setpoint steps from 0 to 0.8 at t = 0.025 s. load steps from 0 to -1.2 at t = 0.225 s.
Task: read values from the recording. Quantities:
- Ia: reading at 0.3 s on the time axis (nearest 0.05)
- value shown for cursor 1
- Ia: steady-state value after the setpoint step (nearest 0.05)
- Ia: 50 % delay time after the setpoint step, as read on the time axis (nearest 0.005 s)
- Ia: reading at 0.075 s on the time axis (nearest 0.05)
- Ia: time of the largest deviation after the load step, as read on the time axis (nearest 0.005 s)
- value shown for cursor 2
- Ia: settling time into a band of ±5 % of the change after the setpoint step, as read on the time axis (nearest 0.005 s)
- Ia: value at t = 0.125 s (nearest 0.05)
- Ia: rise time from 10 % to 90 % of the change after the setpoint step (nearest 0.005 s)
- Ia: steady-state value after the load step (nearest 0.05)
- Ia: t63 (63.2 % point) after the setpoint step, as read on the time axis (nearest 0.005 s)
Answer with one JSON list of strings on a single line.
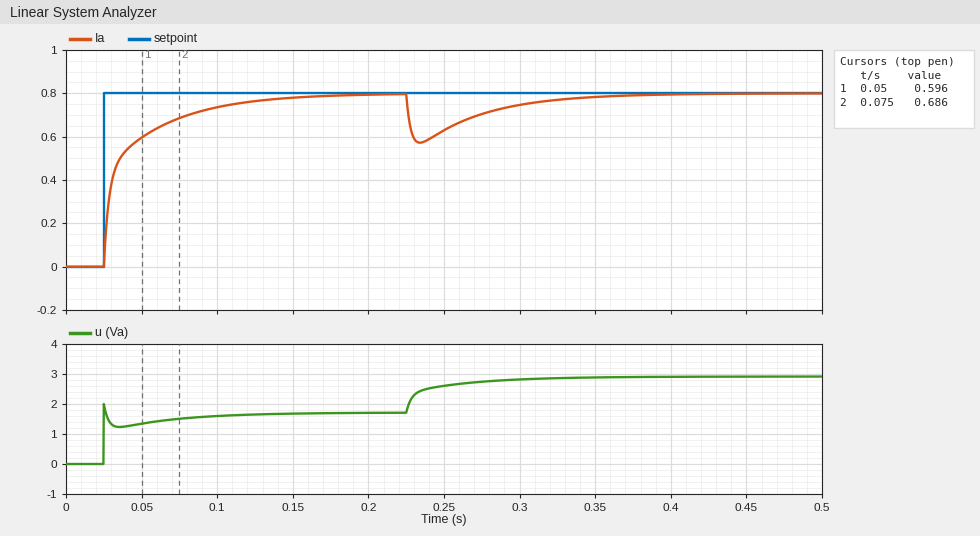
["0.75", "0.596", "0.80", "0.030 s", "0.70", "0.235 s", "0.686", "0.120 s", "0.75", "0.065 s", "0.80", "0.035 s"]
